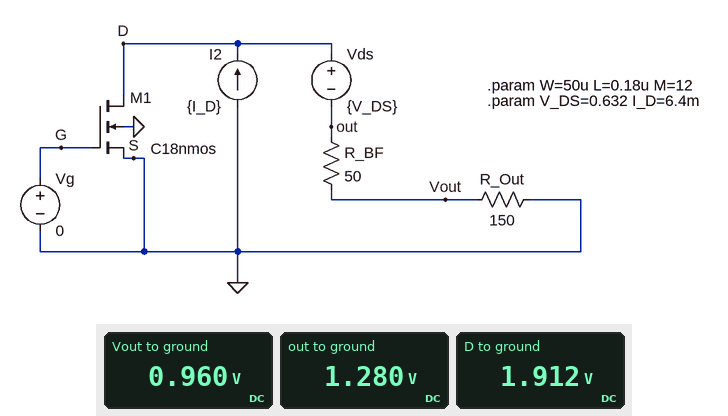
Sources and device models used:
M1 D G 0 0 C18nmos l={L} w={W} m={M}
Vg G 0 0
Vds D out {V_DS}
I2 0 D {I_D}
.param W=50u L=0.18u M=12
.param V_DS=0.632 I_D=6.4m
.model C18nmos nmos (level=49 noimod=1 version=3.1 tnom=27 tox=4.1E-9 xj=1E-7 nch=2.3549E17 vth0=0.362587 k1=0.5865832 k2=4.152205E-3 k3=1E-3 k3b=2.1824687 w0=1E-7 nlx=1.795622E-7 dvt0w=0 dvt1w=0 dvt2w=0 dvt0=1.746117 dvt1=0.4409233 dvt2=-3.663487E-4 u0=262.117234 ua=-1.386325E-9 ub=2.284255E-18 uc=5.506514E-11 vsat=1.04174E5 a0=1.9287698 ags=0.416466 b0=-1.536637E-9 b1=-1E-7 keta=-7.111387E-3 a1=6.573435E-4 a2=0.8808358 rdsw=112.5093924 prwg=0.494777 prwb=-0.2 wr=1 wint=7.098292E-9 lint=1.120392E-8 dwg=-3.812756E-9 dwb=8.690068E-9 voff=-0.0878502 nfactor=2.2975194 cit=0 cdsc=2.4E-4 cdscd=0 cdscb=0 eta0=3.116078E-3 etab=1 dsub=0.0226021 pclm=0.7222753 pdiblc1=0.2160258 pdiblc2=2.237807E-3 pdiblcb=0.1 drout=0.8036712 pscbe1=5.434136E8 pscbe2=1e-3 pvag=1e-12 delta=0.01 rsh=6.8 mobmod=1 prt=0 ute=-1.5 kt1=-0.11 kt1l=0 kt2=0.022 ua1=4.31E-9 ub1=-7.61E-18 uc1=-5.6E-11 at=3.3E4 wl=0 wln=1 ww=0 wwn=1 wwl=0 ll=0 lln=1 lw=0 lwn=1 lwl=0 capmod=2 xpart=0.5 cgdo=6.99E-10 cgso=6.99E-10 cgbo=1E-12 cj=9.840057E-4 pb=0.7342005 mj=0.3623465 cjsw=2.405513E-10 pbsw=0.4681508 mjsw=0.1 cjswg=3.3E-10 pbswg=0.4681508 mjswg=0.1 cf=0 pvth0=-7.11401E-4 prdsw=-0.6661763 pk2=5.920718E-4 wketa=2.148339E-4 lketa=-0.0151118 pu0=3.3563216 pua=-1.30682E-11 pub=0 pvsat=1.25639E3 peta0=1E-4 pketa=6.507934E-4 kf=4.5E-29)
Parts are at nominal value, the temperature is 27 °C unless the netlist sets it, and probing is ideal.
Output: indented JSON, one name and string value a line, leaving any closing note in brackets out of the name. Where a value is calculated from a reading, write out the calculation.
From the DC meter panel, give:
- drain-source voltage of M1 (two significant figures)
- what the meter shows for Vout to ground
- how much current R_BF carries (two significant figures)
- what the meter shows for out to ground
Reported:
{
  "drain-source voltage of M1": "1.912 V = 1.9 V",
  "what the meter shows for Vout to ground": "0.960 V",
  "how much current R_BF carries": "(1.28 V - 960 mV) / 50 Ω = 6.4 mA",
  "what the meter shows for out to ground": "1.280 V"
}
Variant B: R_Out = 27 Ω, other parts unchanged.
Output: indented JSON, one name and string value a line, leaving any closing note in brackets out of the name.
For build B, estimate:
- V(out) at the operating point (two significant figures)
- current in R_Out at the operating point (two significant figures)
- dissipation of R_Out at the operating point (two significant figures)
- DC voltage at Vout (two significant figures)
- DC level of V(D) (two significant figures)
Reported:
{
  "V(out) at the operating point": "490 mV",
  "current in R_Out at the operating point": "6.4 mA",
  "dissipation of R_Out at the operating point": "1.1 mW",
  "DC voltage at Vout": "170 mV",
  "DC level of V(D)": "1.1 V"
}
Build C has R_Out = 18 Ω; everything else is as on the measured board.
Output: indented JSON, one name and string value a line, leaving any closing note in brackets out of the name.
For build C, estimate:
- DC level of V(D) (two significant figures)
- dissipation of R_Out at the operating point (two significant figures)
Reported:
{
  "DC level of V(D)": "1.1 V",
  "dissipation of R_Out at the operating point": "740 µW"
}
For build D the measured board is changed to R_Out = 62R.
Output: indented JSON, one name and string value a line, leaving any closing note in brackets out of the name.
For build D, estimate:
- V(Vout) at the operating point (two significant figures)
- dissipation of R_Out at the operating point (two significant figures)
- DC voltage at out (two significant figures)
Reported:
{
  "V(Vout) at the operating point": "400 mV",
  "dissipation of R_Out at the operating point": "2.5 mW",
  "DC voltage at out": "720 mV"
}
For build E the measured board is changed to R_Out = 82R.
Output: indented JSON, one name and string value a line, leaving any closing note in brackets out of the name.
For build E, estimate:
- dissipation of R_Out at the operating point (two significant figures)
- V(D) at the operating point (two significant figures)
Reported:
{
  "dissipation of R_Out at the operating point": "3.4 mW",
  "V(D) at the operating point": "1.5 V"
}
